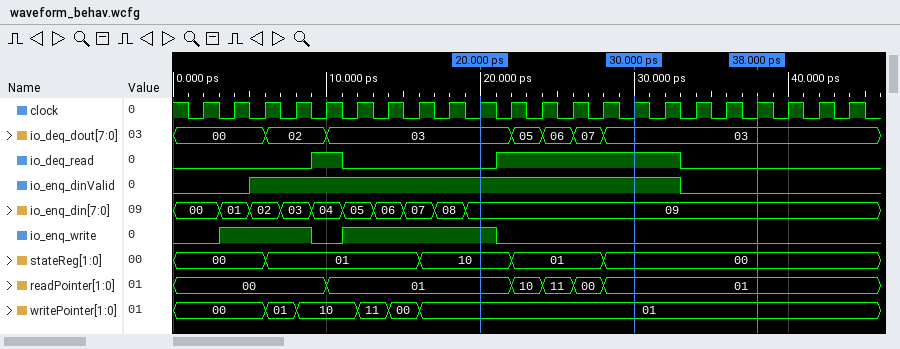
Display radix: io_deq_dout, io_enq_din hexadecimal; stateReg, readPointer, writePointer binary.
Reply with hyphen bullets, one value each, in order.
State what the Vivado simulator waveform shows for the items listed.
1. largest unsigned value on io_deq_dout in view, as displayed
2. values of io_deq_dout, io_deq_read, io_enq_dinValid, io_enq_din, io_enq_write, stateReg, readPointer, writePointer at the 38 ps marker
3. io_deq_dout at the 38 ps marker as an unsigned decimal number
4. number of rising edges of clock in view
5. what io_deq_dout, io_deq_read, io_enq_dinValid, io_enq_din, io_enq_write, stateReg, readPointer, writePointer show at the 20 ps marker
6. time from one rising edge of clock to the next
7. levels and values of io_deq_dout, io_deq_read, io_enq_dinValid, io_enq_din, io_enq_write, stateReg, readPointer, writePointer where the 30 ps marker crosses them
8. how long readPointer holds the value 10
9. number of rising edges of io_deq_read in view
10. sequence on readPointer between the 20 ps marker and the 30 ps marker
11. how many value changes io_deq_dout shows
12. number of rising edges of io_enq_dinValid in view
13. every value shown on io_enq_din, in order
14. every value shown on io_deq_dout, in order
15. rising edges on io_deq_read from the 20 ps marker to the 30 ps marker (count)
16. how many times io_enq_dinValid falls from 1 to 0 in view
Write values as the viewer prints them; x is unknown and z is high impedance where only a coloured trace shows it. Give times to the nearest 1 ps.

- 07
- io_deq_dout=03, io_deq_read=0, io_enq_dinValid=0, io_enq_din=09, io_enq_write=0, stateReg=00, readPointer=01, writePointer=01
- 3
- 22
- io_deq_dout=03, io_deq_read=0, io_enq_dinValid=1, io_enq_din=09, io_enq_write=1, stateReg=10, readPointer=01, writePointer=01
- 2 ps
- io_deq_dout=03, io_deq_read=1, io_enq_dinValid=1, io_enq_din=09, io_enq_write=0, stateReg=00, readPointer=01, writePointer=01
- 2 ps
- 2
- 01, 10, 11, 00, 01
- 6
- 1
- 00, 01, 02, 03, 04, 05, 06, 07, 08, 09
- 00, 02, 03, 05, 06, 07, 03
- 1
- 1
